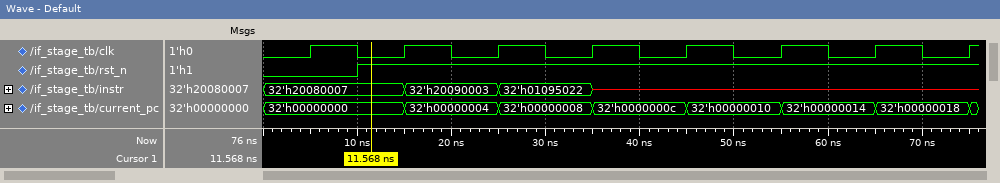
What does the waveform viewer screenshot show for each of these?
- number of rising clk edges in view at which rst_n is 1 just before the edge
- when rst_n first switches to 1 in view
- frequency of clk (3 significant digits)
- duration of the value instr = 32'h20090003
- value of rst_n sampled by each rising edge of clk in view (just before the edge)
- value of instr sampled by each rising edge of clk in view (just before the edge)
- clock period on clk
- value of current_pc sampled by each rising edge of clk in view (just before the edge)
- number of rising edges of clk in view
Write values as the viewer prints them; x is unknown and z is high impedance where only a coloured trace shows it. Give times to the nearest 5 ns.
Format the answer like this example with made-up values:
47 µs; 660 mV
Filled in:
7; 10 ns; 100 MHz; 10 ns; 0 1 1 1 1 1 1 1; 32'h20080007, 32'h20080007, 32'h20090003, 32'h01095022, x, x, x, x; 10 ns; 32'h00000000, 32'h00000000, 32'h00000004, 32'h00000008, 32'h0000000c, 32'h00000010, 32'h00000014, 32'h00000018; 8
